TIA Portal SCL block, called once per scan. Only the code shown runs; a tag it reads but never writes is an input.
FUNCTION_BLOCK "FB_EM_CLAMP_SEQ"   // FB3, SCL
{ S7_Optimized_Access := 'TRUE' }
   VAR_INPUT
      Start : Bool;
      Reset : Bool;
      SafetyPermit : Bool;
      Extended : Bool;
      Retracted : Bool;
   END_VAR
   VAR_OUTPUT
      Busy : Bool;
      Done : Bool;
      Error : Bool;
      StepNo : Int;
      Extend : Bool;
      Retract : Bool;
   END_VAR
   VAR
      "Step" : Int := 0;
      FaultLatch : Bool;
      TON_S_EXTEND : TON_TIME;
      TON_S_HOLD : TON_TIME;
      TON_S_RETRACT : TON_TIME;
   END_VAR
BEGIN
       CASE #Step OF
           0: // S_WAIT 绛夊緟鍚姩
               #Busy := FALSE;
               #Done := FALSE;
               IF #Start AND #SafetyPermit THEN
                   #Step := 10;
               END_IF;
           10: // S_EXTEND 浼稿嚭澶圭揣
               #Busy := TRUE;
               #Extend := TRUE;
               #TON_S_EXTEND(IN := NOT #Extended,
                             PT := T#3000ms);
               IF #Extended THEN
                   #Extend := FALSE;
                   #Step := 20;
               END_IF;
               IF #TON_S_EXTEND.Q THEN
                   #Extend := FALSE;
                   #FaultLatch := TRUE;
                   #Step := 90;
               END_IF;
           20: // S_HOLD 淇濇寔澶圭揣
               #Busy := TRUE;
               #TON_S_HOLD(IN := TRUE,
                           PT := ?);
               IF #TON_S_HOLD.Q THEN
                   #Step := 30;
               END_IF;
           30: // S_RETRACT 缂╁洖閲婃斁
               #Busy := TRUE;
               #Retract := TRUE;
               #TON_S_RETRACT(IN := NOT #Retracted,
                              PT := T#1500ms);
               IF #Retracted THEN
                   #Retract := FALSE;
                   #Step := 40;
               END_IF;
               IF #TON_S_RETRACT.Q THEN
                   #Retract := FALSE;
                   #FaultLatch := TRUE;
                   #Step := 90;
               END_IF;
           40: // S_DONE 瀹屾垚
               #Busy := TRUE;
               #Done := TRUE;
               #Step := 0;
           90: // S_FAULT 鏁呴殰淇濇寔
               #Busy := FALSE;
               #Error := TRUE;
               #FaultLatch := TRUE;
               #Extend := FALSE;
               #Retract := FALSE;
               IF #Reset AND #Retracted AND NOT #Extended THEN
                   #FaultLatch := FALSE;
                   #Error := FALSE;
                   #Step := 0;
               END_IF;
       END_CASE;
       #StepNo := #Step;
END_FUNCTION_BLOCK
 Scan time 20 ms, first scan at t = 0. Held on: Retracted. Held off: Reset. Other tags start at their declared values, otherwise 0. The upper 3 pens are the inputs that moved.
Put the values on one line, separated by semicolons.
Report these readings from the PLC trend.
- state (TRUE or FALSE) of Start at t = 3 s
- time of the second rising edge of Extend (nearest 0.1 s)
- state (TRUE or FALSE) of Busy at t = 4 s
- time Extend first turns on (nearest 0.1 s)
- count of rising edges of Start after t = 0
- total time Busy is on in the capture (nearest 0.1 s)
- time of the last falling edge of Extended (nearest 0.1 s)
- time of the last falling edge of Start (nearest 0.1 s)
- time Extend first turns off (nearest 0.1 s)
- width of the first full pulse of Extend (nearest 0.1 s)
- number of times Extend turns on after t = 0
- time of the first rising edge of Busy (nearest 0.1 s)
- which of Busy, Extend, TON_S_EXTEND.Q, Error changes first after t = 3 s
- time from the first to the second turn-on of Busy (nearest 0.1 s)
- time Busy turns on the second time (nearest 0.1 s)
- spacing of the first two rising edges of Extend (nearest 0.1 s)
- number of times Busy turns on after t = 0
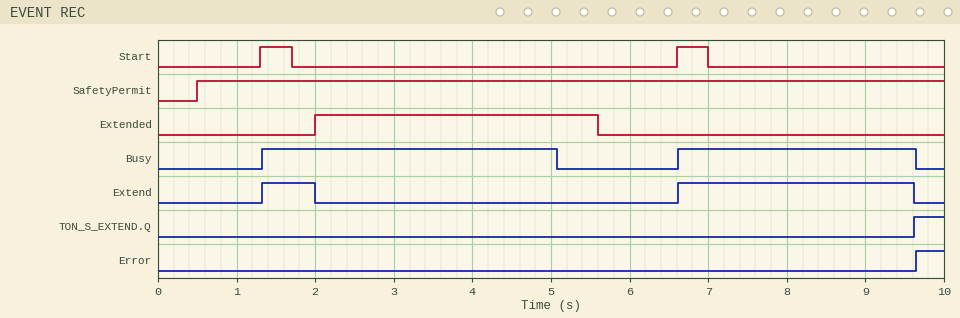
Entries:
FALSE; 6.6 s; TRUE; 1.3 s; 2; 6.8 s; 5.6 s; 7.0 s; 2.0 s; 0.7 s; 2; 1.3 s; Busy; 5.3 s; 6.6 s; 5.3 s; 2
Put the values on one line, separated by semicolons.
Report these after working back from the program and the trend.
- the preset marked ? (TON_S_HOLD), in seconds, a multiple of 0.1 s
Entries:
3.0 s
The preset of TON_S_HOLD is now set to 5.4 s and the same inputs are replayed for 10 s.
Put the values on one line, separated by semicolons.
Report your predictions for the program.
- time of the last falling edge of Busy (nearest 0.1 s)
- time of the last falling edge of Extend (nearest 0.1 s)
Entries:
7.5 s; 2.0 s
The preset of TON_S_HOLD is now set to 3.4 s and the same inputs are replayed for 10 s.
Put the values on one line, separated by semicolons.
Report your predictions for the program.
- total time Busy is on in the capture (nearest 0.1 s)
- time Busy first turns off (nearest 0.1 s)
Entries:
7.2 s; 5.5 s
